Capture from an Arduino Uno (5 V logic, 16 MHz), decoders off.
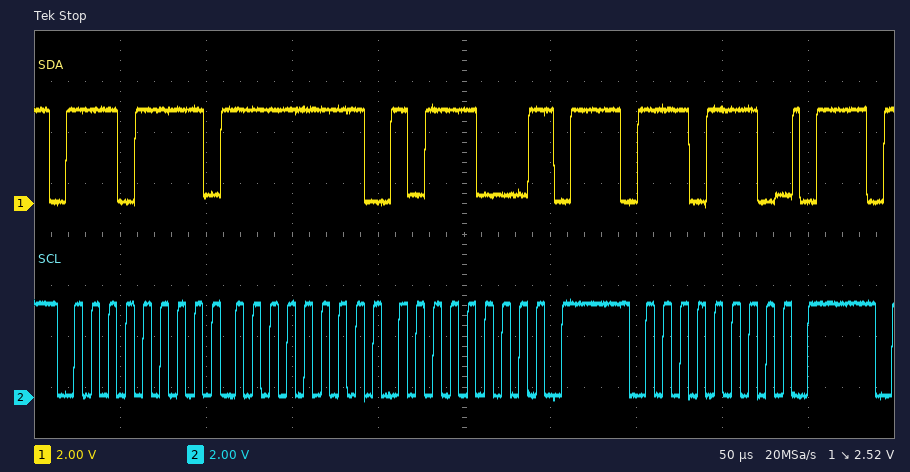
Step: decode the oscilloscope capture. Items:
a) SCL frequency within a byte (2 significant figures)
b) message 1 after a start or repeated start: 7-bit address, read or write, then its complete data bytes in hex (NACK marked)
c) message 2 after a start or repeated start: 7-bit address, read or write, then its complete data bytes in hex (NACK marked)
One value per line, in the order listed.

100 kHz
0x77 read: FF B8 NACK
0x77 write
